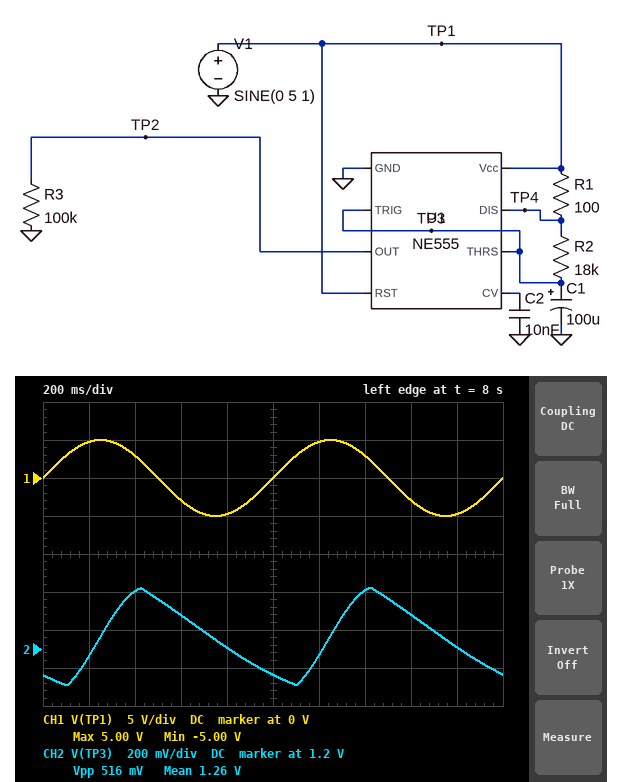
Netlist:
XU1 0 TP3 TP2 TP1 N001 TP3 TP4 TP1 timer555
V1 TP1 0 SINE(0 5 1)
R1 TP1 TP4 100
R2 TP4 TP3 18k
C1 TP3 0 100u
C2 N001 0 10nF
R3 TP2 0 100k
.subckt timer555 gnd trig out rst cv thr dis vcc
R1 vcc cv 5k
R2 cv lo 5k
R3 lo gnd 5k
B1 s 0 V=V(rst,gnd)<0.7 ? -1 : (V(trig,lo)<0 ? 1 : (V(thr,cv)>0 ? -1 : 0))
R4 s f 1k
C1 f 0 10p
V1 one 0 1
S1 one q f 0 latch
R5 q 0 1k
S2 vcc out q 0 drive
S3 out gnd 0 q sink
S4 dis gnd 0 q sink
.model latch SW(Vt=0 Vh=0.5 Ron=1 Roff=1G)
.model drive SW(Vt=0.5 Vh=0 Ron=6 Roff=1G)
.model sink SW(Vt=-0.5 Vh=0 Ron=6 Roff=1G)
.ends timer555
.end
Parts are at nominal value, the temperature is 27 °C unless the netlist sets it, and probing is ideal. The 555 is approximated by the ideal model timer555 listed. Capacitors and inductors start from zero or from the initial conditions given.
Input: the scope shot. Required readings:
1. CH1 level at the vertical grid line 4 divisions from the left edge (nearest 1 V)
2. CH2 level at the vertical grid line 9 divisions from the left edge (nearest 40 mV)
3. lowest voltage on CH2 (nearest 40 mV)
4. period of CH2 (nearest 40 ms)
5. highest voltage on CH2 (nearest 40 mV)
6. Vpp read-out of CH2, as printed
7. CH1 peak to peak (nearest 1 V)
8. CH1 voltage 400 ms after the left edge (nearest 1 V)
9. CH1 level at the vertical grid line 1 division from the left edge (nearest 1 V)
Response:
-5 V
1.20 V
1.00 V
1.00 s
1.52 V
516 mV
10 V
3 V
5 V
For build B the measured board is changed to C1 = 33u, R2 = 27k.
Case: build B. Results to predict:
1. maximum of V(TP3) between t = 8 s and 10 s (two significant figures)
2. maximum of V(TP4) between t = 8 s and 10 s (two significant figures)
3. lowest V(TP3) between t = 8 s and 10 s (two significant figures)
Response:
1.8 V
5.0 V
800 mV
